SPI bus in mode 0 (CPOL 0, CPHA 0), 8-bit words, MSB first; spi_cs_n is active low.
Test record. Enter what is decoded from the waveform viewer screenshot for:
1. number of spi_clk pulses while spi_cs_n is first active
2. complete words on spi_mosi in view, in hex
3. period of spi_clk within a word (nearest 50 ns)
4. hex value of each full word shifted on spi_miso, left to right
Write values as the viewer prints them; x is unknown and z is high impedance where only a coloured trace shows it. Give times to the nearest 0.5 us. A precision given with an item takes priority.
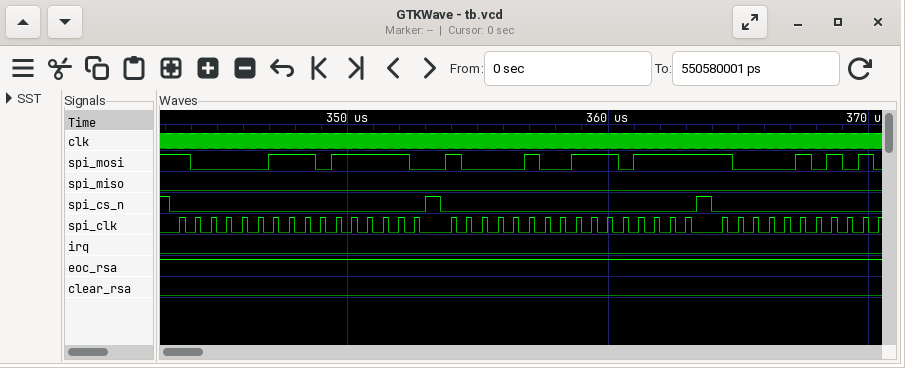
16
83, BE, 84, EF, 85
600 ns
00, 00, 00, 00, 00
